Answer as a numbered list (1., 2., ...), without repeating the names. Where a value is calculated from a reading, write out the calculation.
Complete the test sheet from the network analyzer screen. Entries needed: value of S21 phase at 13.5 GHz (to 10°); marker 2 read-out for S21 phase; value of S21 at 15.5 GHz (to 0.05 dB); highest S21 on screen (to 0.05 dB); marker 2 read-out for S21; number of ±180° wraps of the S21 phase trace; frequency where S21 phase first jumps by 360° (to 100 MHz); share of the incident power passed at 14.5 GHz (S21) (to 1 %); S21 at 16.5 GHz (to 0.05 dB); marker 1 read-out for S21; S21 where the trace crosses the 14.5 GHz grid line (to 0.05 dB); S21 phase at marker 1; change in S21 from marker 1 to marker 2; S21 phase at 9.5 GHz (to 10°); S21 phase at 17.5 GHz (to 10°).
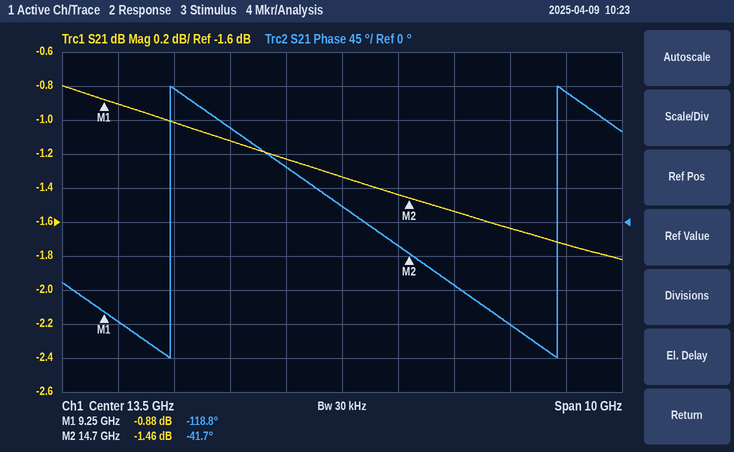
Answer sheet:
1. 20°
2. -41.7°
3. -1.55 dB
4. -0.80 dB
5. -1.46 dB
6. 2
7. 10.4 GHz
8. 10^(-1.45/10) ≈ 72 %
9. -1.65 dB
10. -0.88 dB
11. -1.45 dB
12. -118.8°
13. -1.46 − (-0.88) = -0.58 dB
14. -130°
15. 170°
